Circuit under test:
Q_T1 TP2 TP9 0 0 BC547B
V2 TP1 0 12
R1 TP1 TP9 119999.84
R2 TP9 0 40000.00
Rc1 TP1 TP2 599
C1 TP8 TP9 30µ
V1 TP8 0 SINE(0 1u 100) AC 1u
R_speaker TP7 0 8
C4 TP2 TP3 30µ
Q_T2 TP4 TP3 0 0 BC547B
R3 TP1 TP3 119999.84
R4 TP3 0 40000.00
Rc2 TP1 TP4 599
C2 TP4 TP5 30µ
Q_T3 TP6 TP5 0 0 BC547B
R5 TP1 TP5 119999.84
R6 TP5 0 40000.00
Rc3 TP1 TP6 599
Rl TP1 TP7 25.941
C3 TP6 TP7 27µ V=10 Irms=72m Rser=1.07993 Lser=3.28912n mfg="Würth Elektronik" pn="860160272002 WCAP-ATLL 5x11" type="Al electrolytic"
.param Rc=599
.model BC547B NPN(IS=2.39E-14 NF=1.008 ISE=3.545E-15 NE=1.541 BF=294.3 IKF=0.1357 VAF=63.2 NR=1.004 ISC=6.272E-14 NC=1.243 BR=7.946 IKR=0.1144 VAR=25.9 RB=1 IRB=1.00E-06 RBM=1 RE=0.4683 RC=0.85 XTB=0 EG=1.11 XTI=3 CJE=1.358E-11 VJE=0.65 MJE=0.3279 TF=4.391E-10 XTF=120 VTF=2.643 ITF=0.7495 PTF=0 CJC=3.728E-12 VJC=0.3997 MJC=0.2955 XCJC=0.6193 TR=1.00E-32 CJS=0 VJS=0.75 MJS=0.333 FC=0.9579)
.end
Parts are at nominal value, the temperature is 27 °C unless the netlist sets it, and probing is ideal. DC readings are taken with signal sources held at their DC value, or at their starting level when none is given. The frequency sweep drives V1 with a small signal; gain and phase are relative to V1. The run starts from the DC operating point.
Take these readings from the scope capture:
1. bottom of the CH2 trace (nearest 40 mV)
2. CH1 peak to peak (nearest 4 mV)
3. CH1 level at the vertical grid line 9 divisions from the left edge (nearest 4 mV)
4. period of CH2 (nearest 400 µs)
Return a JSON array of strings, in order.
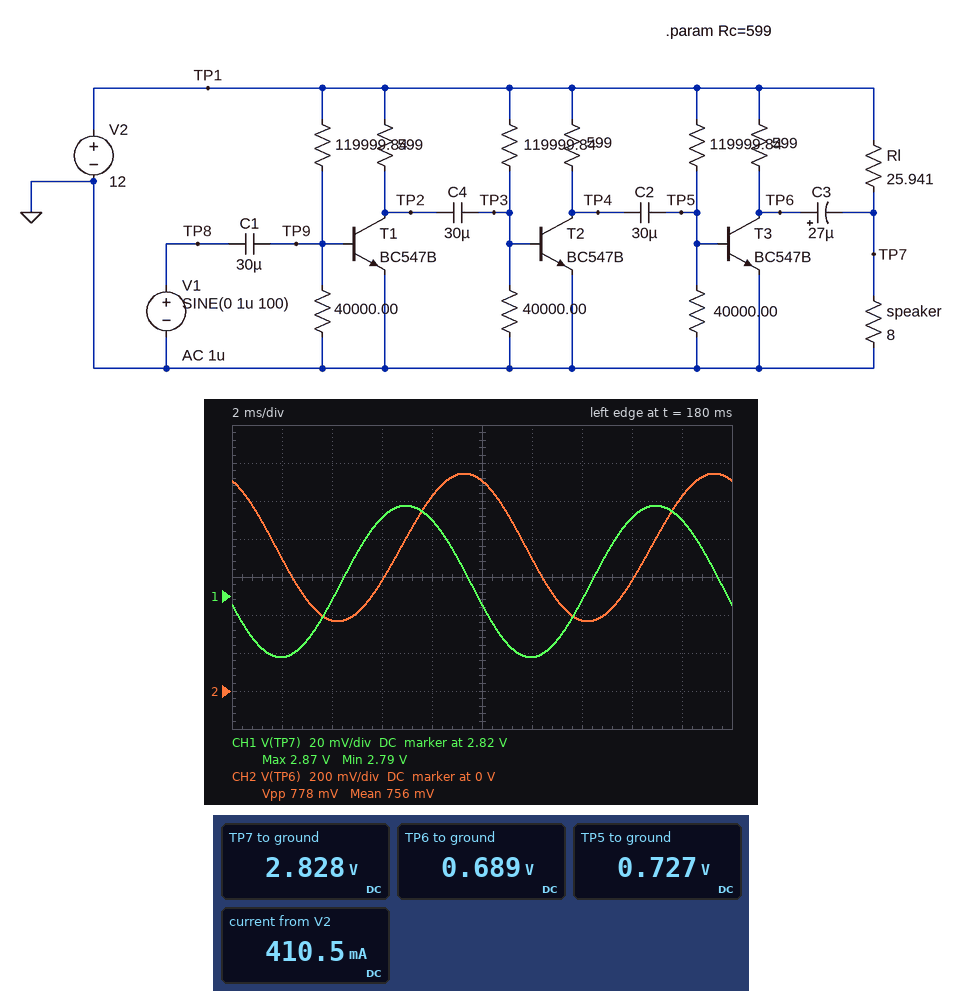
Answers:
["360 mV", "80 mV", "2.860 V", "10.0 ms"]
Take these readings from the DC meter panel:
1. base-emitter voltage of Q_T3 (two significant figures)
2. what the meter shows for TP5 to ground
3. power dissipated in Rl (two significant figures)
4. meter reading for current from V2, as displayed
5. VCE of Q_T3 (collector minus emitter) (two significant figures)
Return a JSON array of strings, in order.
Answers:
["730 mV", "0.727 V", "3.2 W", "410.5 mA", "690 mV"]
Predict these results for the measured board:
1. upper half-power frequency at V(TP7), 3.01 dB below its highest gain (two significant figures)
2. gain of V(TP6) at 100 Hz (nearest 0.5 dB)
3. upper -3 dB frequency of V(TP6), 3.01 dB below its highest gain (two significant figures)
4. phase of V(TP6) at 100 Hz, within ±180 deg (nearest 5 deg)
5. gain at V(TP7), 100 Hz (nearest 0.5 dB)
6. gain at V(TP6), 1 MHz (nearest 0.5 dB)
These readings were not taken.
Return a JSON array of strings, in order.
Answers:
["610 kHz", "112.0 dB", "34 Hz", "115 deg", "92.0 dB", "88.0 dB"]
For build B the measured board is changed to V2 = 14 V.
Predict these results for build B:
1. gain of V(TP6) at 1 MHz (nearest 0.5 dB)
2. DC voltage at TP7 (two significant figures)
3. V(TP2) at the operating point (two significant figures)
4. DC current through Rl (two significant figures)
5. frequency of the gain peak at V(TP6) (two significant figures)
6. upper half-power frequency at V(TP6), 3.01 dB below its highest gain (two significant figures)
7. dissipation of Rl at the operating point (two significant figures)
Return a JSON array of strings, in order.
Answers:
["88.5 dB", "3.3 V", "580 mV", "410 mA", "16 Hz", "37 Hz", "4.4 W"]
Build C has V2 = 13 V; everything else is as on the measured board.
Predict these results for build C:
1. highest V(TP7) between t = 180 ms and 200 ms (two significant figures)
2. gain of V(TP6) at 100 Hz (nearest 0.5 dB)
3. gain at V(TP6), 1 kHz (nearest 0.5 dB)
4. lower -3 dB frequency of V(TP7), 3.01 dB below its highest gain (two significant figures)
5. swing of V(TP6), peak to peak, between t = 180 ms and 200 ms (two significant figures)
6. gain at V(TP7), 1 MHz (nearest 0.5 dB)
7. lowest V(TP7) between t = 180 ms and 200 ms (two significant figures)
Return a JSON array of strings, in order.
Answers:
["3.1 V", "112.5 dB", "96.5 dB", "22 Hz", "840 mV", "87.0 dB", "3.0 V"]
